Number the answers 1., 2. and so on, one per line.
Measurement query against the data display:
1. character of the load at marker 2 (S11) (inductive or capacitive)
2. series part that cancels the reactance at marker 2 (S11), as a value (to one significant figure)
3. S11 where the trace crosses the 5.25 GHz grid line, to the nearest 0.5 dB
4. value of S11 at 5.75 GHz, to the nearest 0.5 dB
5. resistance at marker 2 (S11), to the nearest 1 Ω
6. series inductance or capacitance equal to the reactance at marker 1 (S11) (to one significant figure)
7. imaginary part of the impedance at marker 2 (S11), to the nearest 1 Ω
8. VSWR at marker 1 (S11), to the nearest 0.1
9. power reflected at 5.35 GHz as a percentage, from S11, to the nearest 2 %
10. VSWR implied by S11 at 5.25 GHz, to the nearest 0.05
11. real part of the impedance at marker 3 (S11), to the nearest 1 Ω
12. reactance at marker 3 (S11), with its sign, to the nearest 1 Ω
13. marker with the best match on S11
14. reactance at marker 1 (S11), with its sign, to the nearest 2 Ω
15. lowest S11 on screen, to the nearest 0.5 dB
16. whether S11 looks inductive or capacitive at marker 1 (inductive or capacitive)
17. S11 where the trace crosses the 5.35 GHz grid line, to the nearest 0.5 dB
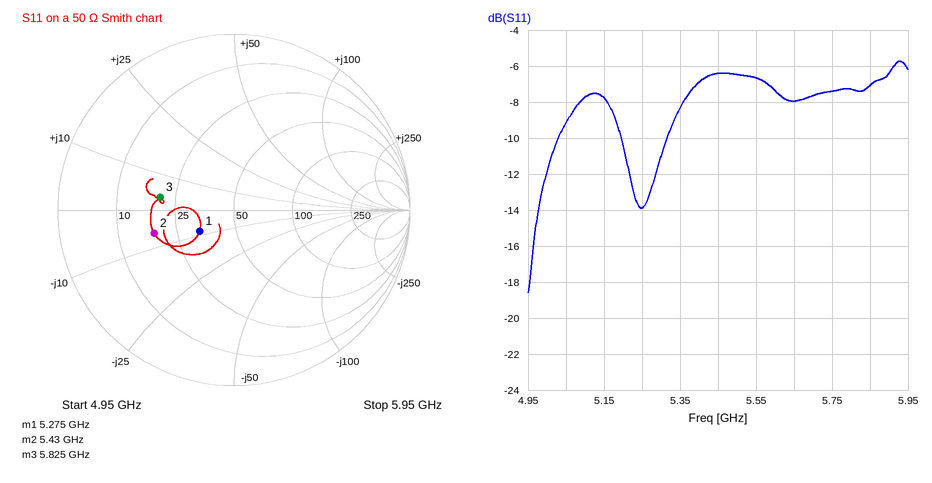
1. capacitive
2. 200 pH
3. -14.0 dB
4. -7.5 dB
5. 18 Ω
6. 4 pF
7. -6 Ω
8. 1.6
9. 14 %
10. 1.50
11. 20 Ω
12. +4 Ω
13. marker 1
14. -8 Ω
15. -18.5 dB
16. capacitive
17. -8.5 dB
